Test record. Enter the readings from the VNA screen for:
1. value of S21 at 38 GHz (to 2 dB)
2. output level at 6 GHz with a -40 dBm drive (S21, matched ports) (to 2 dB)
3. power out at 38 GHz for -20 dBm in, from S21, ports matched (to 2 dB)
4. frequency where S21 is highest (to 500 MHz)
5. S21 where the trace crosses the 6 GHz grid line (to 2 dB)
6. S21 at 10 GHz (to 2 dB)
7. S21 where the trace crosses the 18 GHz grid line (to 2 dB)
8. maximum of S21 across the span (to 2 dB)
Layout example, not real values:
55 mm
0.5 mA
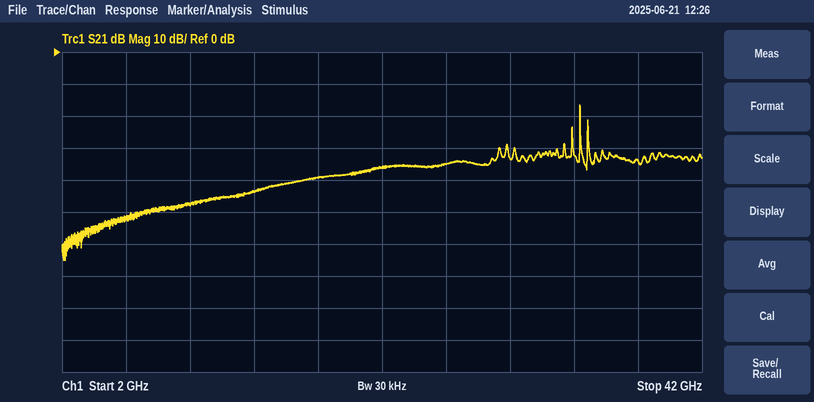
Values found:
-34 dB
-92 dBm
-54 dBm
34.5 GHz
-52 dB
-48 dB
-40 dB
-16 dB
